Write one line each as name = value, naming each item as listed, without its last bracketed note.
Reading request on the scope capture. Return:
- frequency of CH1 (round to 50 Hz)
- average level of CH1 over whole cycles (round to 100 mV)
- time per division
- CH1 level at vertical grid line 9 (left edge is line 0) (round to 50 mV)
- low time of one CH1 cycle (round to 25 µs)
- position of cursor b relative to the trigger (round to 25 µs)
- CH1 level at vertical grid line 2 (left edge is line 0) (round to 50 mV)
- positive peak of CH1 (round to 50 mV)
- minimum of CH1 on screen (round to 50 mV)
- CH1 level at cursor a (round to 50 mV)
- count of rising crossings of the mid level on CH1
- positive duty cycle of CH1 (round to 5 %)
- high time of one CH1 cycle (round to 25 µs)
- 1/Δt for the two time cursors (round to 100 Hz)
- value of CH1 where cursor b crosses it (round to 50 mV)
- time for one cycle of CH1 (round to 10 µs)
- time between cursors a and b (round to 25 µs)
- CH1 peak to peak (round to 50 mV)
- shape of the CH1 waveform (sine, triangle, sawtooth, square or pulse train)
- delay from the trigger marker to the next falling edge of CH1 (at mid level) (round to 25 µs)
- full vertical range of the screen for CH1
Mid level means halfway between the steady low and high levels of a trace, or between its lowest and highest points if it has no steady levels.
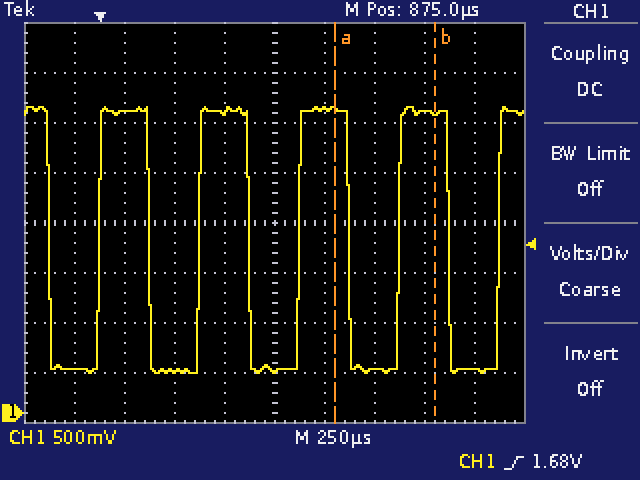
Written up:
frequency of CH1 = 2.00 kHz
average level of CH1 over whole cycles = 1.7 V
time per division = 250 µs
CH1 level at vertical grid line 9 (left edge is line 0) = 450 mV
low time of one CH1 cycle = 250 µs
position of cursor b relative to the trigger = +1.675 ms
CH1 level at vertical grid line 2 (left edge is line 0) = 3.00 V
positive peak of CH1 = 3.05 V
minimum of CH1 on screen = 400 mV
CH1 level at cursor a = 3.05 V
count of rising crossings of the mid level on CH1 = 5
positive duty cycle of CH1 = 50 %
high time of one CH1 cycle = 250 µs
1/Δt for the two time cursors = 2.0 kHz
value of CH1 where cursor b crosses it = 3.00 V
time for one cycle of CH1 = 500 µs
time between cursors a and b = 500 µs
CH1 peak to peak = 2.65 V
shape of the CH1 waveform = square
delay from the trigger marker to the next falling edge of CH1 (at mid level) = 250 µs
full vertical range of the screen for CH1 = 4 V
